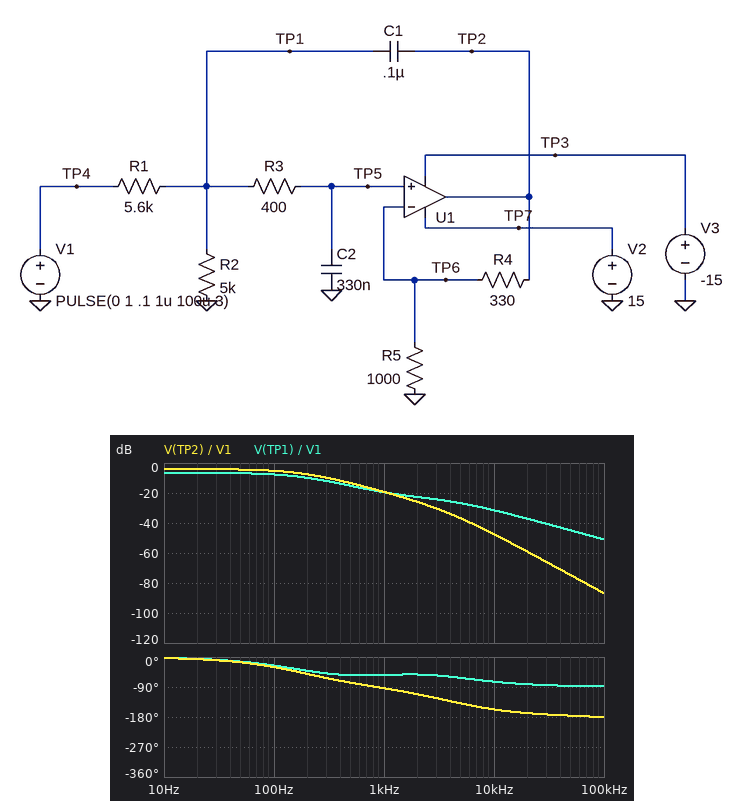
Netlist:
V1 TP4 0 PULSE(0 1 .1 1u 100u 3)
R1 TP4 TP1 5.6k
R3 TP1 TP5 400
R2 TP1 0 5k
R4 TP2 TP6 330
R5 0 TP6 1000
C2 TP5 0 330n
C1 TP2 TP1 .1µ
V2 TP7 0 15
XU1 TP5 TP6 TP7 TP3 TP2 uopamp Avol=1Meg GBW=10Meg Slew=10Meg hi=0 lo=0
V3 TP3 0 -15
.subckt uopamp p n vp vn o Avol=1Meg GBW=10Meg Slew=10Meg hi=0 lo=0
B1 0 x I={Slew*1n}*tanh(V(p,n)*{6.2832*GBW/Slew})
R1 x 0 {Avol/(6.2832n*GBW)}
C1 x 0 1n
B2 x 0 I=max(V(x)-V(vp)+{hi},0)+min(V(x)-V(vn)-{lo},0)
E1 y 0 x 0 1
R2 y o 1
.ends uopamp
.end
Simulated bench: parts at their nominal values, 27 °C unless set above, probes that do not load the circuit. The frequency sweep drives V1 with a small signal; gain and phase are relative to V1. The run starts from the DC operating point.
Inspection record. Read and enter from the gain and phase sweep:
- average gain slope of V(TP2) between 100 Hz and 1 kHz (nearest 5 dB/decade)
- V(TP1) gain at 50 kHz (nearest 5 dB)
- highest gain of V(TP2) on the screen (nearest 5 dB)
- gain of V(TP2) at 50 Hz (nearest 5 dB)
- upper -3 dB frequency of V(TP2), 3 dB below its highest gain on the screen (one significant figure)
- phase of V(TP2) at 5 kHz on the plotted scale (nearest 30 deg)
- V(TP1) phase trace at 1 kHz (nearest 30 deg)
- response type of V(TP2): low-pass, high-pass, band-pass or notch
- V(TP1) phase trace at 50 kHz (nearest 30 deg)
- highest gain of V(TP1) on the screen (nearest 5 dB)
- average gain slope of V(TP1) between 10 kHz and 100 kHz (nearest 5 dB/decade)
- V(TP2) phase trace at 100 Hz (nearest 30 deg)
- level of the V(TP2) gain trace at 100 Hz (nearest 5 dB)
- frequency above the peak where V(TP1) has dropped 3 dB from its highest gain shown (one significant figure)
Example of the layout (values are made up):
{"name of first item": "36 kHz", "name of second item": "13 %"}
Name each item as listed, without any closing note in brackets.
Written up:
{"average gain slope of V(TP2) between 100 Hz and 1 kHz": "-15 dB/decade", "V(TP1) gain at 50 kHz": "-45 dB", "highest gain of V(TP2) on the screen": "-5 dB", "gain of V(TP2) at 50 Hz": "-5 dB", "upper -3 dB frequency of V(TP2), 3 dB below its highest gain on the screen": "200 Hz", "phase of V(TP2) at 5 kHz on the plotted scale": "-150 deg", "V(TP1) phase trace at 1 kHz": "-60 deg", "response type of V(TP2): low-pass, high-pass, band-pass or notch": "low-pass", "V(TP1) phase trace at 50 kHz": "-90 deg", "highest gain of V(TP1) on the screen": "-5 dB", "average gain slope of V(TP1) between 10 kHz and 100 kHz": "-20 dB/decade", "V(TP2) phase trace at 100 Hz": "-30 deg", "level of the V(TP2) gain trace at 100 Hz": "-5 dB", "frequency above the peak where V(TP1) has dropped 3 dB from its highest gain shown": "200 Hz"}
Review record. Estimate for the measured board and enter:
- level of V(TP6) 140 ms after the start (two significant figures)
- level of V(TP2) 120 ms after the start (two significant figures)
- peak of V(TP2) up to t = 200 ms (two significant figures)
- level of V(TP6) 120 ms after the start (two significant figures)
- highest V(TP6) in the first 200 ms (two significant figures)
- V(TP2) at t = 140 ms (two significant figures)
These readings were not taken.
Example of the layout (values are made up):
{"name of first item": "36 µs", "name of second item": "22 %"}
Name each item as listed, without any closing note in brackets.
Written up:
{"level of V(TP6) 140 ms after the start": "470 mV", "level of V(TP2) 120 ms after the start": "630 mV", "peak of V(TP2) up to t = 200 ms": "630 mV", "level of V(TP6) 120 ms after the start": "470 mV", "highest V(TP6) in the first 200 ms": "470 mV", "V(TP2) at t = 140 ms": "630 mV"}
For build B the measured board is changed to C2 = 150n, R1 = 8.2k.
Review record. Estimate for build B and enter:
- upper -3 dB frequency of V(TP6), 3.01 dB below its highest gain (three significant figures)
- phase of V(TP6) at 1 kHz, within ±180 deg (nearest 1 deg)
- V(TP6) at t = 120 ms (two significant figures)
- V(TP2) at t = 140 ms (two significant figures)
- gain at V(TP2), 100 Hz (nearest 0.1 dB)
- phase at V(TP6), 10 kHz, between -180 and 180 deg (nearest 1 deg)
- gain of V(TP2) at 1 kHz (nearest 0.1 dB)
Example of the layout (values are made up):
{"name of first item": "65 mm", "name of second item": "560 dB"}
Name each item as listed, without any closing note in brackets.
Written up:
{"upper -3 dB frequency of V(TP6), 3.01 dB below its highest gain": "419 Hz", "phase of V(TP6) at 1 kHz, within ±180 deg": "-84 deg", "V(TP6) at t = 120 ms": "380 mV", "V(TP2) at t = 140 ms": "500 mV", "gain at V(TP2), 100 Hz": "-6.2 dB", "phase at V(TP6), 10 kHz, between -180 and 180 deg": "-160 deg", "gain of V(TP2) at 1 kHz": "-14.5 dB"}
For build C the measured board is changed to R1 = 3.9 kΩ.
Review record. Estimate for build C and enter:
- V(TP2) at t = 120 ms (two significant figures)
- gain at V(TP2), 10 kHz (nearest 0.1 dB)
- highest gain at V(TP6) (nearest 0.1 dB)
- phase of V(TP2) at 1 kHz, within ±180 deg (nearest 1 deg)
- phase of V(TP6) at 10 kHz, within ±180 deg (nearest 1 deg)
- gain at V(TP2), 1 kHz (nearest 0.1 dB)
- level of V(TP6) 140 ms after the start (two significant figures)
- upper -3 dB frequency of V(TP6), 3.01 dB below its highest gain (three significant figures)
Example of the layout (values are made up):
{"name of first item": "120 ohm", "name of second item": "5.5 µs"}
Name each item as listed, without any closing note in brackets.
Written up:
{"V(TP2) at t = 120 ms": "750 mV", "gain at V(TP2), 10 kHz": "-44.4 dB", "highest gain at V(TP6)": "-5.0 dB", "phase of V(TP2) at 1 kHz, within ±180 deg": "-92 deg", "phase of V(TP6) at 10 kHz, within ±180 deg": "-157 deg", "gain at V(TP2), 1 kHz": "-16.4 dB", "level of V(TP6) 140 ms after the start": "560 mV", "upper -3 dB frequency of V(TP6), 3.01 dB below its highest gain": "213 Hz"}
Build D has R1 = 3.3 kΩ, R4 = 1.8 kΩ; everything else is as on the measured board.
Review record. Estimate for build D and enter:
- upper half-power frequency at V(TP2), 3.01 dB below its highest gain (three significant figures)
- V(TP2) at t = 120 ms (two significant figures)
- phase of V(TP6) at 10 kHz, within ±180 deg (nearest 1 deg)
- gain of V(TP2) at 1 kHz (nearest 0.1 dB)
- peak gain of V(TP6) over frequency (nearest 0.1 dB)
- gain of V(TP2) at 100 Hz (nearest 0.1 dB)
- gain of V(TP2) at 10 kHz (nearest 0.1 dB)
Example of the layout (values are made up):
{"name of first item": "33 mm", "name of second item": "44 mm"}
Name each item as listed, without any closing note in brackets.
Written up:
{"upper half-power frequency at V(TP2), 3.01 dB below its highest gain": "429 Hz", "V(TP2) at t = 120 ms": "1.7 V", "phase of V(TP6) at 10 kHz, within ±180 deg": "-165 deg", "gain of V(TP2) at 1 kHz": "-4.1 dB", "peak gain of V(TP6) over frequency": "-4.4 dB", "gain of V(TP2) at 100 Hz": "4.3 dB", "gain of V(TP2) at 10 kHz": "-36.0 dB"}
